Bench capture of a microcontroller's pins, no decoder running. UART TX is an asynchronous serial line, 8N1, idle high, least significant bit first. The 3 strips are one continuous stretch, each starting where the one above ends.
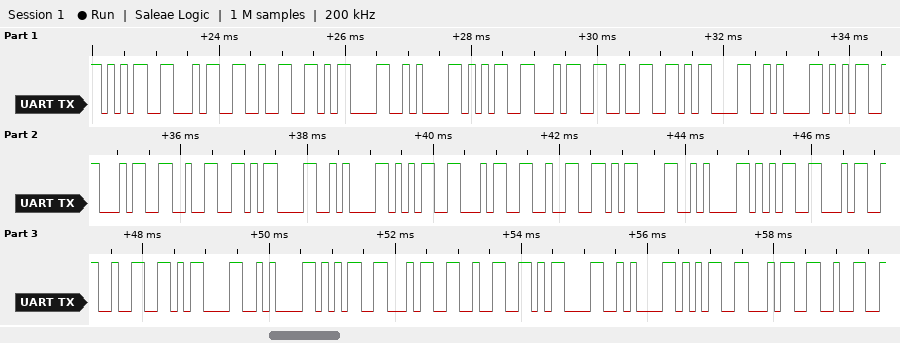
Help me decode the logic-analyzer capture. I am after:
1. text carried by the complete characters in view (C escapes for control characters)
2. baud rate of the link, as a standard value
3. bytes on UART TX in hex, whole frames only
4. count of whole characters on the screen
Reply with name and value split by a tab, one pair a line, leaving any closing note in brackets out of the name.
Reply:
text carried by the complete characters in view	"542\r\n542\r\n542\r\n542\r\n542\r\n542\r\n542"
baud rate of the link, as a standard value	9600 baud
bytes on UART TX in hex, whole frames only	35 34 32 0D 0A 35 34 32 0D 0A 35 34 32 0D 0A 35 34 32 0D 0A 35 34 32 0D 0A 35 34 32 0D 0A 35 34 32
count of whole characters on the screen	33
